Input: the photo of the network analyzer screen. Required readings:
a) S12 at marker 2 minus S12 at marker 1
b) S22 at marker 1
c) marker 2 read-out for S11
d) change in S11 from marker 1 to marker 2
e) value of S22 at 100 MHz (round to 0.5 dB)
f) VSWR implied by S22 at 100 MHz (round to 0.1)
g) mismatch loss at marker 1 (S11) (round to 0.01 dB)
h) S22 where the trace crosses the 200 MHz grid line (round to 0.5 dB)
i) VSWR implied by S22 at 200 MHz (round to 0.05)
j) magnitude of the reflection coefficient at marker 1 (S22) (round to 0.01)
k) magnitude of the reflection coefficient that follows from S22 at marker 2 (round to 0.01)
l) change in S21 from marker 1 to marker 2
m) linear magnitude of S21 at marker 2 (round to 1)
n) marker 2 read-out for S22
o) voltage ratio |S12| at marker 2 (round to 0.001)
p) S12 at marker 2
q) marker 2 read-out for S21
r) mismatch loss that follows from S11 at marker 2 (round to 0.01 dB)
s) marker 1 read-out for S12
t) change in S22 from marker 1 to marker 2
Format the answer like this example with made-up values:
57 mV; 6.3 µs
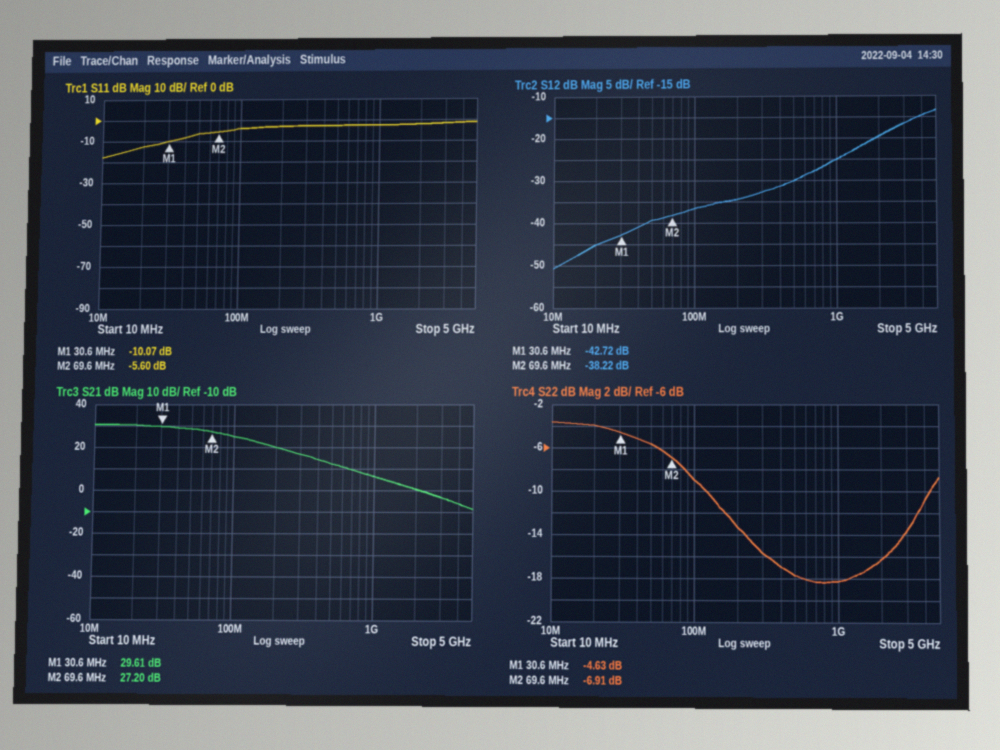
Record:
4.50 dB; -4.63 dB; -5.60 dB; 4.47 dB; -9.0 dB; 2.1; 0.45 dB; -13.5 dB; 1.55; 0.59; 0.45; -2.41 dB; 23; -6.91 dB; 0.012; -38.22 dB; 27.20 dB; 1.40 dB; -42.72 dB; -2.28 dB
